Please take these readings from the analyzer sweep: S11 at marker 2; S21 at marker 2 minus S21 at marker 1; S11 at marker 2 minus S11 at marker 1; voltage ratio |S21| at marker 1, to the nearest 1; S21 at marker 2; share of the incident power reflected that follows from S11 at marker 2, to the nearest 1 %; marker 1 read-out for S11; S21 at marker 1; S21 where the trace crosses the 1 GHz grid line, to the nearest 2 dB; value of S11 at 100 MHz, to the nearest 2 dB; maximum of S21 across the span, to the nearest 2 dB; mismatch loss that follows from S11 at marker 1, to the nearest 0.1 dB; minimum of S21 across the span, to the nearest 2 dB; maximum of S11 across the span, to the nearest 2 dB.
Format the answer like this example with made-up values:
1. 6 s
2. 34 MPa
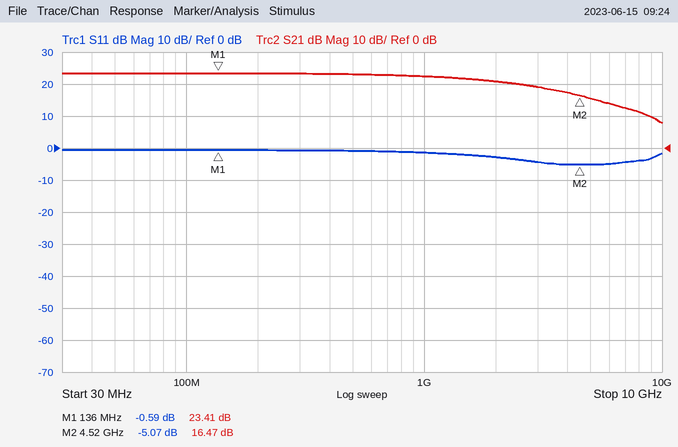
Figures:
1. -5.07 dB
2. -6.94 dB
3. -4.48 dB
4. 15
5. 16.47 dB
6. 31 %
7. -0.59 dB
8. 23.41 dB
9. 22 dB
10. 0 dB
11. 24 dB
12. 9.0 dB
13. 8 dB
14. 0 dB
